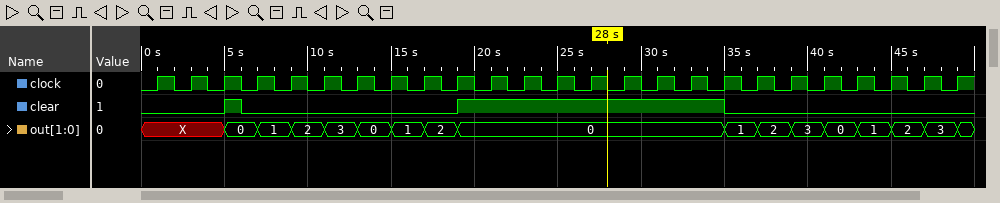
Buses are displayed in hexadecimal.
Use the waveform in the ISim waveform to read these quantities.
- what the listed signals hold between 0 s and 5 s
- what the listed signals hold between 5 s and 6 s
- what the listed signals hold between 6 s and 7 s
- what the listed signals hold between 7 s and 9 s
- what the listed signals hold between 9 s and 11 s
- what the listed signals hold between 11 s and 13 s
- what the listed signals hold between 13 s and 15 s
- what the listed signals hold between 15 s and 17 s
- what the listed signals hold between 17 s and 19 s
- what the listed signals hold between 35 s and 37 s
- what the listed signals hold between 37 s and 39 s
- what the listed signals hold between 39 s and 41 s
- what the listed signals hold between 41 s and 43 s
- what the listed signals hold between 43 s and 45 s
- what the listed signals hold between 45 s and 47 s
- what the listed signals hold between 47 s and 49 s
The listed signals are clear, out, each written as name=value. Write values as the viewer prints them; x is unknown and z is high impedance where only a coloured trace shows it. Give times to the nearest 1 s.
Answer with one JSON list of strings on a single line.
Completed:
["clear=0, out=X", "clear=1, out=0", "clear=0, out=0", "clear=0, out=1", "clear=0, out=2", "clear=0, out=3", "clear=0, out=0", "clear=0, out=1", "clear=0, out=2", "clear=0, out=1", "clear=0, out=2", "clear=0, out=3", "clear=0, out=0", "clear=0, out=1", "clear=0, out=2", "clear=0, out=3"]
